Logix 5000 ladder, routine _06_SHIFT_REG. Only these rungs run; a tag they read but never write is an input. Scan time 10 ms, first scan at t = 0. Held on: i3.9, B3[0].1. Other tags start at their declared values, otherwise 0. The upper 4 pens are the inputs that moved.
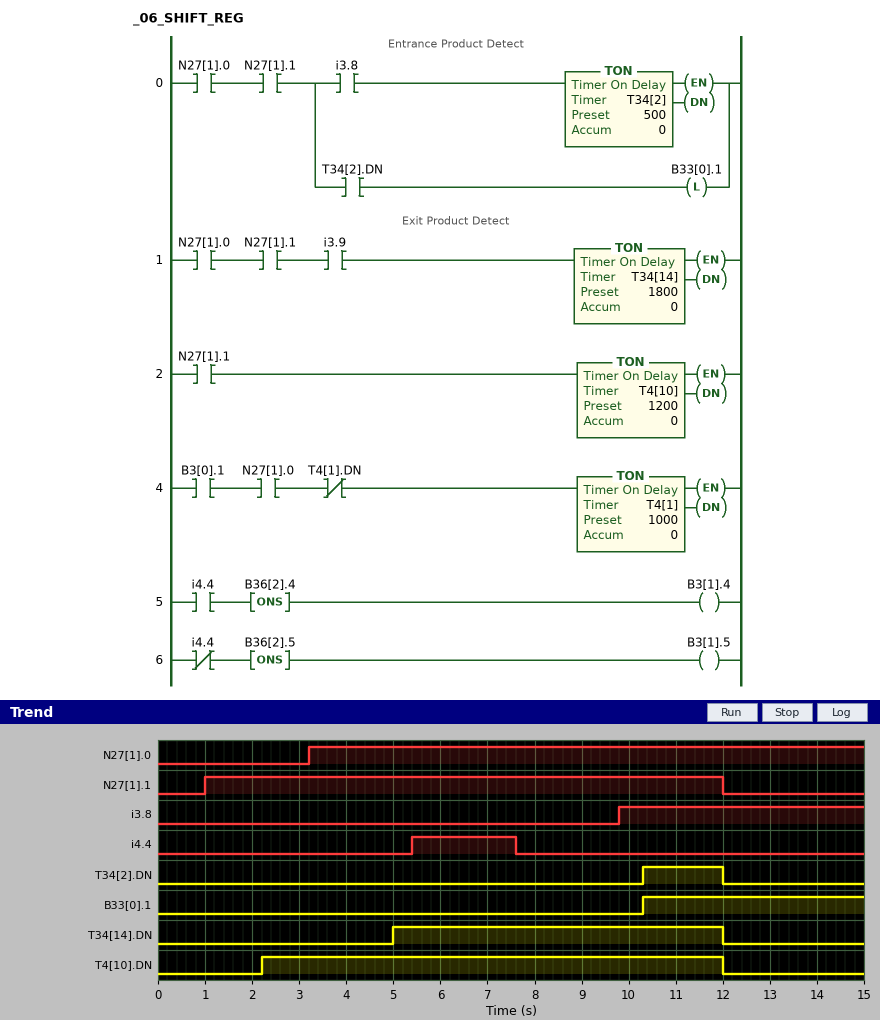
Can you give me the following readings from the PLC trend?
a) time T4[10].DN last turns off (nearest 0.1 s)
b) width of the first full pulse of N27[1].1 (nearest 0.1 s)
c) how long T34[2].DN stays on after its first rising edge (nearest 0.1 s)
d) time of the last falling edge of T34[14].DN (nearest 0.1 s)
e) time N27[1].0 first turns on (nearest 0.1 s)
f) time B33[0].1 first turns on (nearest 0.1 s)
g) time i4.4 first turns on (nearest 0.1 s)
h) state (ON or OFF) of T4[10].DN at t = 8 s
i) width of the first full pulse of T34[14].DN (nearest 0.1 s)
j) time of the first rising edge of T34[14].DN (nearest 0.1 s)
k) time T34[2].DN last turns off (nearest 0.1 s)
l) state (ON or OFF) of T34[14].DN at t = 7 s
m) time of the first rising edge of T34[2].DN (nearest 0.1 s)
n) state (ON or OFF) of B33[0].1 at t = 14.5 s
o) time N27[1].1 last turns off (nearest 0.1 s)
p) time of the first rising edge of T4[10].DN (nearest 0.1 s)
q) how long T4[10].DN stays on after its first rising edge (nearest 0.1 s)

12.0 s
11.0 s
1.7 s
12.0 s
3.2 s
10.3 s
5.4 s
ON
7.0 s
5.0 s
12.0 s
ON
10.3 s
ON
12.0 s
2.2 s
9.8 s
